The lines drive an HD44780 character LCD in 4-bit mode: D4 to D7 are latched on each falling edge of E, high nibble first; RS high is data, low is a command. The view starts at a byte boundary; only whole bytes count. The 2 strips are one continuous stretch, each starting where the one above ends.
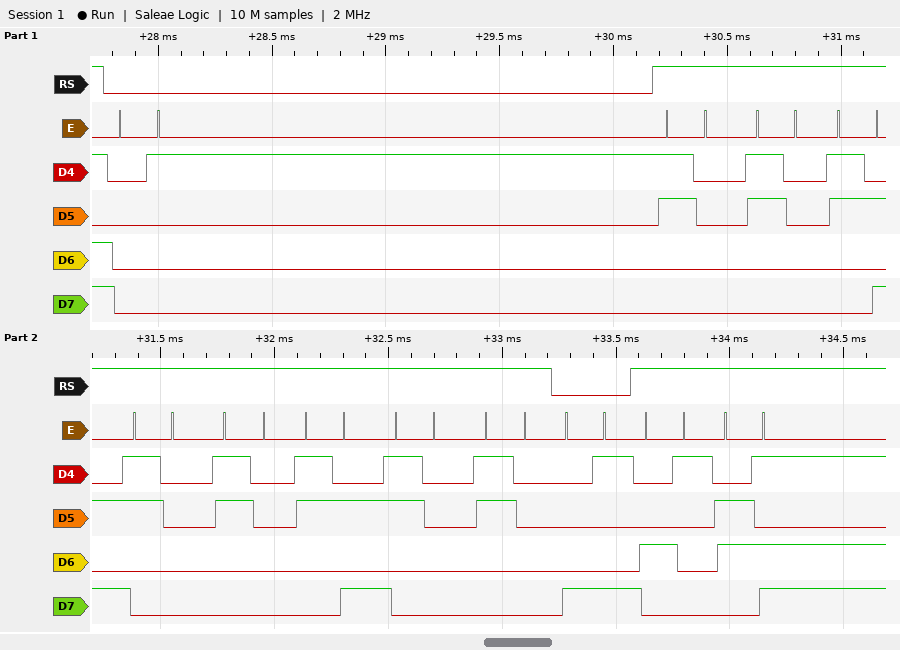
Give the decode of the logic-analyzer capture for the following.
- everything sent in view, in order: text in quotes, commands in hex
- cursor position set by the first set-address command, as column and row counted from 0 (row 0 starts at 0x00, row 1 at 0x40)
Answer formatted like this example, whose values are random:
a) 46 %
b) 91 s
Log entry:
a) 0x01 "00:00:00" 0x89 "Am"
b) column 9, row 0
